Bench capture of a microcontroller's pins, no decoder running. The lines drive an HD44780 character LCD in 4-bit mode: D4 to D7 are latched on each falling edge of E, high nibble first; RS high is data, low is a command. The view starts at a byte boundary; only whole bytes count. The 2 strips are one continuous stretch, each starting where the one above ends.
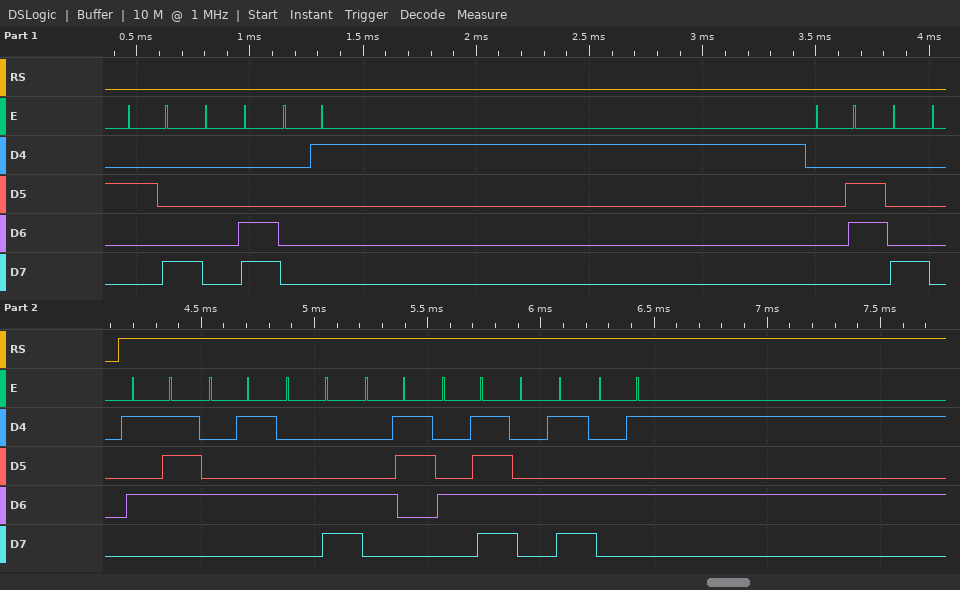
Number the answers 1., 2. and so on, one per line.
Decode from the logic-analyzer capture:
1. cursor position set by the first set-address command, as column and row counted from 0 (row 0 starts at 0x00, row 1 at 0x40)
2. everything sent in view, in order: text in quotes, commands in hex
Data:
1. column 0, row 0
2. 0x28 0x0C 0x01 0x06 0x80 "WELCOME"
